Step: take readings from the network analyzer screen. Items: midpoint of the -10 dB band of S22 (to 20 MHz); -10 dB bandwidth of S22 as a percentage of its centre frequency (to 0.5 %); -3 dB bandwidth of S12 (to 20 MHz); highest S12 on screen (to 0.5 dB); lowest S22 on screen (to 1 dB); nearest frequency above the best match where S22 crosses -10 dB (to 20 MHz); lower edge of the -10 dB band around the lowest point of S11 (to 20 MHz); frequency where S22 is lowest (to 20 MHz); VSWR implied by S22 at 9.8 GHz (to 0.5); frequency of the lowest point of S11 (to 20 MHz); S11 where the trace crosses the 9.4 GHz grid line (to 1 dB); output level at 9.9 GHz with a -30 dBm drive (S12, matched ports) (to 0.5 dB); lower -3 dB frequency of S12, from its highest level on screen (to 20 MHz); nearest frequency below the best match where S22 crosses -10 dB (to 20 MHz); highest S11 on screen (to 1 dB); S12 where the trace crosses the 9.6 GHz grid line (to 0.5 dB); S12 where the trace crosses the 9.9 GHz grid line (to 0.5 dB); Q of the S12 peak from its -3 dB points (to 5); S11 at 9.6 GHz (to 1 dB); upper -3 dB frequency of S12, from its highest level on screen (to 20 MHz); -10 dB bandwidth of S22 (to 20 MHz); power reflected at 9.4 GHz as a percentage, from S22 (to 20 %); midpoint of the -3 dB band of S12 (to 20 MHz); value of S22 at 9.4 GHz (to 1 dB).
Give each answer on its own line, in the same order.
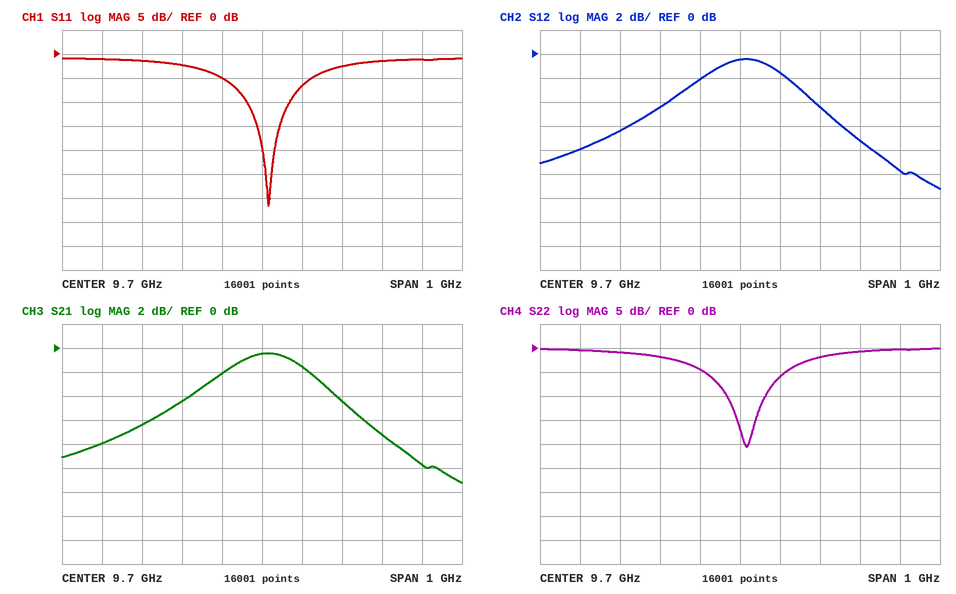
9.72 GHz
1.0 %
320 MHz
-0.5 dB
-21 dB
9.76 GHz
9.66 GHz
9.72 GHz
3.0
9.72 GHz
-1 dB
-34.5 dBm
9.54 GHz
9.66 GHz
-1 dB
-2.0 dB
-4.5 dB
30
-5 dB
9.86 GHz
100 MHz
80 %
9.70 GHz
-1 dB
